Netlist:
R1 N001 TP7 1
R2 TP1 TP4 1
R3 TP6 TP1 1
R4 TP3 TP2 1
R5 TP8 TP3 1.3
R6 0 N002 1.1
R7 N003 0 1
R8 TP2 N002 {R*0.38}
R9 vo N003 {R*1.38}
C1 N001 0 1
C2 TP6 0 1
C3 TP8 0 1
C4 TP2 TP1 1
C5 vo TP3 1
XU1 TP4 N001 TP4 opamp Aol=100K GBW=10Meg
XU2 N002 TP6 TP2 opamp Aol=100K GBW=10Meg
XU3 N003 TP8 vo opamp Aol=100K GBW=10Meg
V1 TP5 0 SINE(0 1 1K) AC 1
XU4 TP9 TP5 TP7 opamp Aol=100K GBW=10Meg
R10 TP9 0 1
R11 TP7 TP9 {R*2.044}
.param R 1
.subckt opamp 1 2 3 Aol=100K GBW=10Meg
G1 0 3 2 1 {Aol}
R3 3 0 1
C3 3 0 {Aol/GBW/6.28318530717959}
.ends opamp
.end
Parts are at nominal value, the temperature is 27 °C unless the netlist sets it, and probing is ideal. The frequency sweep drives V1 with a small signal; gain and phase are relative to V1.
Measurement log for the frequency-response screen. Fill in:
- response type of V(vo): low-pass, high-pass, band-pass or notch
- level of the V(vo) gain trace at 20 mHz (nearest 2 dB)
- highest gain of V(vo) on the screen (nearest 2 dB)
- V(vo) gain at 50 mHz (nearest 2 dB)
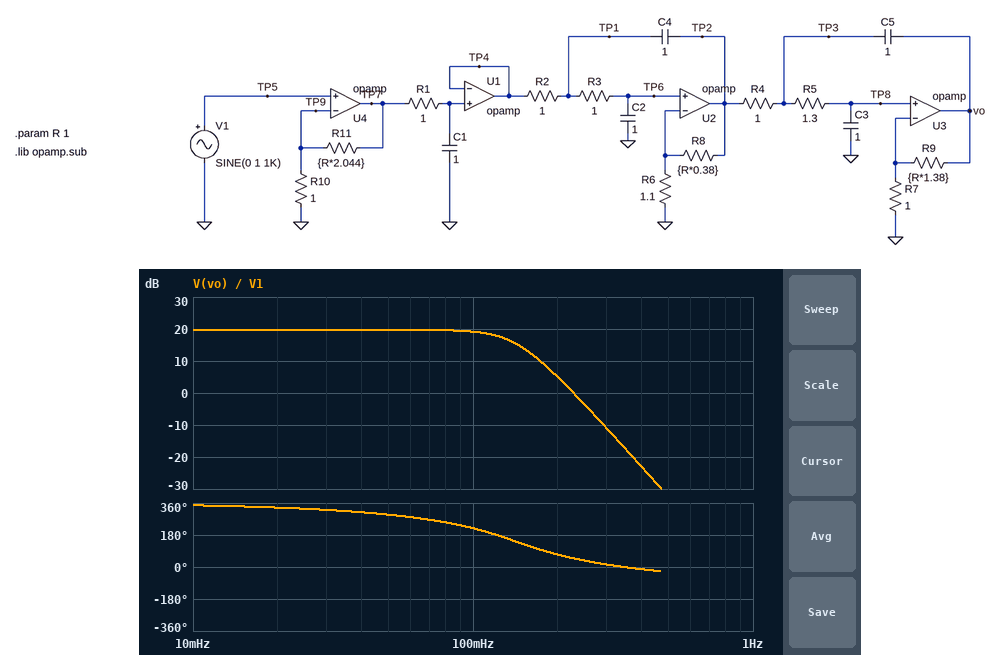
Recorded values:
low-pass
20 dB
20 dB
20 dB
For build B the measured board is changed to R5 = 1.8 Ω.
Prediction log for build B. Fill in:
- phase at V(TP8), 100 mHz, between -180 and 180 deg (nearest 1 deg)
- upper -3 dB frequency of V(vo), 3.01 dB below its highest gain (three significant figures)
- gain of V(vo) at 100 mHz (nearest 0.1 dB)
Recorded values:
-164 deg
105 mHz
17.3 dB
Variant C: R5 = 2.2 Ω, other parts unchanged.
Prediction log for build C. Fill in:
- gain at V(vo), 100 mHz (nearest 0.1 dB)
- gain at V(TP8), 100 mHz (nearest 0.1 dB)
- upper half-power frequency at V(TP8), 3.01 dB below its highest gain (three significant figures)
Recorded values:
15.5 dB
8.0 dB
89.5 mHz
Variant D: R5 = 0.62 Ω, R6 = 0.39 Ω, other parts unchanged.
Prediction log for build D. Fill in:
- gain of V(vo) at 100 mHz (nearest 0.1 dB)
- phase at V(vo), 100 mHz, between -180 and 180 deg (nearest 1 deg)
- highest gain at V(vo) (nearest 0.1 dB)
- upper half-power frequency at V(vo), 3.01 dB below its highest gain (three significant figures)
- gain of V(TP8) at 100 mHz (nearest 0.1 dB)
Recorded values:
25.0 dB
-90 deg
27.3 dB
212 mHz
17.5 dB
